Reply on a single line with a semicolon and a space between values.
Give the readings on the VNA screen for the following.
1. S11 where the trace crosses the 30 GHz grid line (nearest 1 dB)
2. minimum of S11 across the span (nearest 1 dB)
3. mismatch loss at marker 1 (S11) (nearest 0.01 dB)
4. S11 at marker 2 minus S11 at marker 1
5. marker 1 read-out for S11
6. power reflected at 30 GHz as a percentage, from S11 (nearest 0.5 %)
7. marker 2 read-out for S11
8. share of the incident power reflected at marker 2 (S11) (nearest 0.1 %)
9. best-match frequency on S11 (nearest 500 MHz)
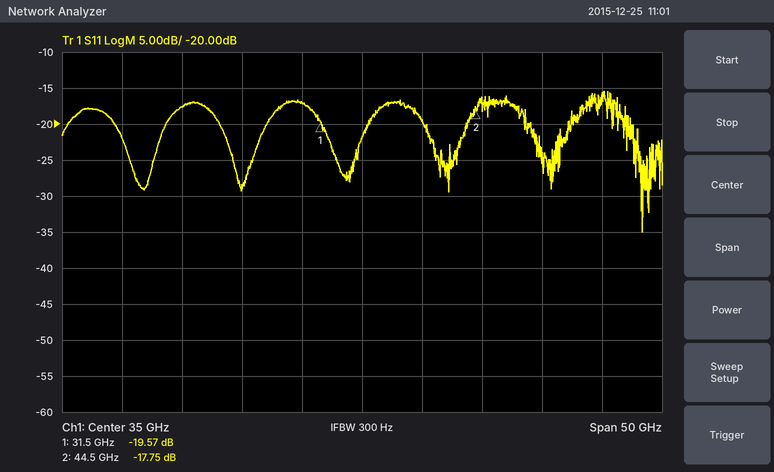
-17 dB; -35 dB; 0.05 dB; 1.82 dB; -19.57 dB; 2.0 %; -17.75 dB; 1.7 %; 58.5 GHz
